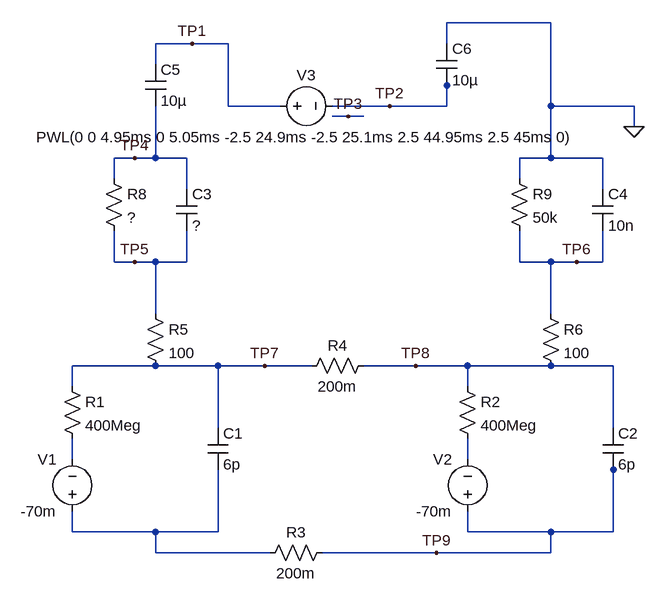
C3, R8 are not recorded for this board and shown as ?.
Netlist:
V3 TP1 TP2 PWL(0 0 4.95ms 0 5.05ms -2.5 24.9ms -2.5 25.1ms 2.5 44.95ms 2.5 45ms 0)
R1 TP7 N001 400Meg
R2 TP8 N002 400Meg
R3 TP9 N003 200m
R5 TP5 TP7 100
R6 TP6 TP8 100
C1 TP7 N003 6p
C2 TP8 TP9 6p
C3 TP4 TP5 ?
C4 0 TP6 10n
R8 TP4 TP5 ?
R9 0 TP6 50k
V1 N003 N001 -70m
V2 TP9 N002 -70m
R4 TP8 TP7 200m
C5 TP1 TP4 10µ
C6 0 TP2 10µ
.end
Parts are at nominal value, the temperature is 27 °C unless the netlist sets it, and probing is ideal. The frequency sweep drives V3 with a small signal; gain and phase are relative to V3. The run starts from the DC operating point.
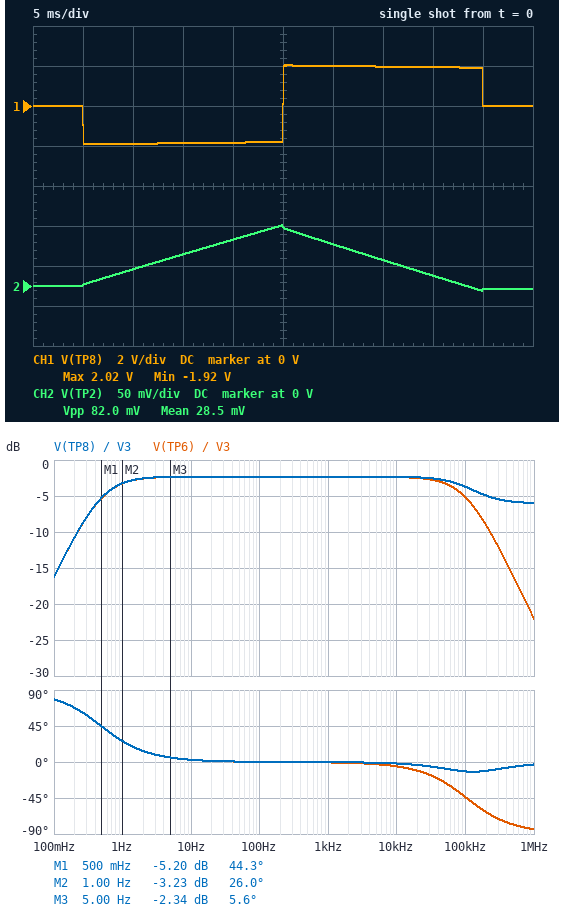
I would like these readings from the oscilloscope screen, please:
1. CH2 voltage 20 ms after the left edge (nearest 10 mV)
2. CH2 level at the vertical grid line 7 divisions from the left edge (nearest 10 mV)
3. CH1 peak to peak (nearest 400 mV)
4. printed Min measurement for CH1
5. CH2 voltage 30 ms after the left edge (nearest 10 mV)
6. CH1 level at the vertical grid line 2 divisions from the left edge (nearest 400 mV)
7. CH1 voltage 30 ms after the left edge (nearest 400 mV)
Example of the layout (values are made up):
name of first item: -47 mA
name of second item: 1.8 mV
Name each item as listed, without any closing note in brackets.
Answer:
CH2 voltage 20 ms after the left edge: 60 mV
CH2 level at the vertical grid line 7 divisions from the left edge: 30 mV
CH1 peak to peak: 4.0 V
printed Min measurement for CH1: -1.92 V
CH2 voltage 30 ms after the left edge: 50 mV
CH1 level at the vertical grid line 2 divisions from the left edge: -2.0 V
CH1 voltage 30 ms after the left edge: 2.0 V
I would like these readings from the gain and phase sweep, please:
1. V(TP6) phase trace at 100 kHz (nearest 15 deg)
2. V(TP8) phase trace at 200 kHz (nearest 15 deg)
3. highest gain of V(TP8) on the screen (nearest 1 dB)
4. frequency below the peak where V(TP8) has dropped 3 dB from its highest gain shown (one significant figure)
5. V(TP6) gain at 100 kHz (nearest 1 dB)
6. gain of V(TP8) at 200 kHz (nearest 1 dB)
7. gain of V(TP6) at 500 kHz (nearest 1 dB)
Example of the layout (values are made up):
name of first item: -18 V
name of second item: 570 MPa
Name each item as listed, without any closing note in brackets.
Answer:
V(TP6) phase trace at 100 kHz: -45 deg
V(TP8) phase trace at 200 kHz: -15 deg
highest gain of V(TP8) on the screen: -2 dB
frequency below the peak where V(TP8) has dropped 3 dB from its highest gain shown: 500 mHz
V(TP6) gain at 100 kHz: -5 dB
gain of V(TP8) at 200 kHz: -5 dB
gain of V(TP6) at 500 kHz: -16 dB
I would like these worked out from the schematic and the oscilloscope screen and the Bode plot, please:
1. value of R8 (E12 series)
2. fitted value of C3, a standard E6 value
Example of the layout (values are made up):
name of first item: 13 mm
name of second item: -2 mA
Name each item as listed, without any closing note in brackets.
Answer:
value of R8: 15 kΩ
fitted value of C3, a standard E6 value: 33 nF
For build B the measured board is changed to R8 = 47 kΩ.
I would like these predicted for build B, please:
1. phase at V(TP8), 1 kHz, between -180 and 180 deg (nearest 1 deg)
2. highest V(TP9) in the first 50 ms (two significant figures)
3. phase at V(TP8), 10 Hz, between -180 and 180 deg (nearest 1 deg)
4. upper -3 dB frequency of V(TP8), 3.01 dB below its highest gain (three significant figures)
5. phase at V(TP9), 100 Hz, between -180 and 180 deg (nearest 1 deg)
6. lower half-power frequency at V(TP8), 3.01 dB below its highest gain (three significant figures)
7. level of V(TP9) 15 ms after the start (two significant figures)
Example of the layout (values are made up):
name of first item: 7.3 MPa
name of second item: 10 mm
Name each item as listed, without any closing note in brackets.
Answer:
phase at V(TP8), 1 kHz, between -180 and 180 deg: 3 deg
highest V(TP9) in the first 50 ms: 2.4 V
phase at V(TP8), 10 Hz, between -180 and 180 deg: 4 deg
upper -3 dB frequency of V(TP8), 3.01 dB below its highest gain: 271 kHz
phase at V(TP9), 100 Hz, between -180 and 180 deg: 11 deg
lower half-power frequency at V(TP8), 3.01 dB below its highest gain: 47.3 Hz
level of V(TP9) 15 ms after the start: -1.3 V
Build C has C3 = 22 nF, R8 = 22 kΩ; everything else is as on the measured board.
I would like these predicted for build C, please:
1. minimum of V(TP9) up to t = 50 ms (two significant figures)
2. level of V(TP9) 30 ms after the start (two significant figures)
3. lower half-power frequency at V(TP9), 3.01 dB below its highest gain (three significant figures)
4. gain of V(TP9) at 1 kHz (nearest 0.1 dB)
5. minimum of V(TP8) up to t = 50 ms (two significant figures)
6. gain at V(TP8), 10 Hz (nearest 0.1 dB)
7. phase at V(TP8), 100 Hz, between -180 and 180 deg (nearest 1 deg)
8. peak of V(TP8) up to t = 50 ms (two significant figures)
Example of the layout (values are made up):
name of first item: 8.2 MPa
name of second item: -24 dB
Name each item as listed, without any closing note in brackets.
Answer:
minimum of V(TP9) up to t = 50 ms: -1.8 V
level of V(TP9) 30 ms after the start: 1.7 V
lower half-power frequency at V(TP9), 3.01 dB below its highest gain: 440 mHz
gain of V(TP9) at 1 kHz: -3.3 dB
minimum of V(TP8) up to t = 50 ms: -1.7 V
gain at V(TP8), 10 Hz: -3.2 dB
phase at V(TP8), 100 Hz, between -180 and 180 deg: 0 deg
peak of V(TP8) up to t = 50 ms: 1.8 V
